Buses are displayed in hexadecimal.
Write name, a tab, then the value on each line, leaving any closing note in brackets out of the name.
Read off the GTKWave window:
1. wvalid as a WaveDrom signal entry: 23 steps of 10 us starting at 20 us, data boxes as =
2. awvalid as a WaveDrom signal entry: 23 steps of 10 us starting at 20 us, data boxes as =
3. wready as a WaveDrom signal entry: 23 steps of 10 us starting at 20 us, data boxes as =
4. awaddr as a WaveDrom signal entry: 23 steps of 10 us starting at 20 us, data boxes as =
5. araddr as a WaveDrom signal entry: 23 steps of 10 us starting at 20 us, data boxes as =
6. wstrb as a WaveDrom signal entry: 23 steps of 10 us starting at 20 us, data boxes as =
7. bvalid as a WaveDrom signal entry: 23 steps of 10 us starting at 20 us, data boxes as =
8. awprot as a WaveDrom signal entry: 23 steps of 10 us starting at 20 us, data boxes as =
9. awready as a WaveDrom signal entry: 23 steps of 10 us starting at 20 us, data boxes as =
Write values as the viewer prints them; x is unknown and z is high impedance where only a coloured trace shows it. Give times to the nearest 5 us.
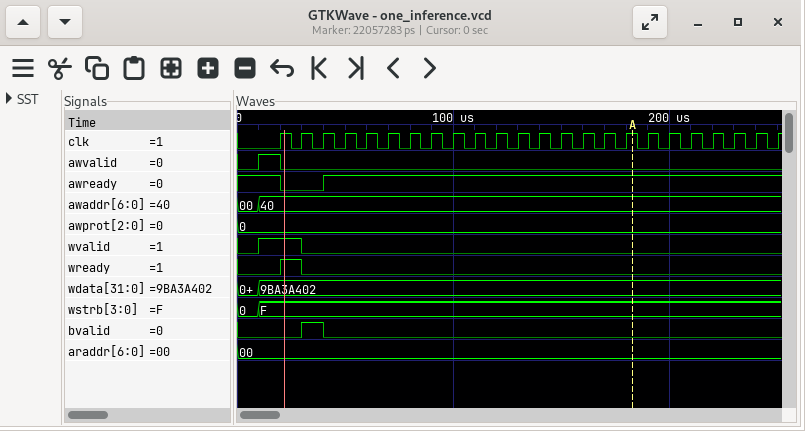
wvalid as a WaveDrom signal entry: 23 steps of 10 us starting at 20 us, data boxes as =	{name: 'wvalid', wave: '10.....................'}
awvalid as a WaveDrom signal entry: 23 steps of 10 us starting at 20 us, data boxes as =	{name: 'awvalid', wave: '0......................'}
wready as a WaveDrom signal entry: 23 steps of 10 us starting at 20 us, data boxes as =	{name: 'wready', wave: '10.....................'}
awaddr as a WaveDrom signal entry: 23 steps of 10 us starting at 20 us, data boxes as =	{name: 'awaddr', wave: '=......................', data: '40'}
araddr as a WaveDrom signal entry: 23 steps of 10 us starting at 20 us, data boxes as =	{name: 'araddr', wave: '=......................', data: '00'}
wstrb as a WaveDrom signal entry: 23 steps of 10 us starting at 20 us, data boxes as =	{name: 'wstrb', wave: '=......................', data: 'F'}
bvalid as a WaveDrom signal entry: 23 steps of 10 us starting at 20 us, data boxes as =	{name: 'bvalid', wave: '010....................'}
awprot as a WaveDrom signal entry: 23 steps of 10 us starting at 20 us, data boxes as =	{name: 'awprot', wave: '=......................', data: '0'}
awready as a WaveDrom signal entry: 23 steps of 10 us starting at 20 us, data boxes as =	{name: 'awready', wave: '0.1....................'}
